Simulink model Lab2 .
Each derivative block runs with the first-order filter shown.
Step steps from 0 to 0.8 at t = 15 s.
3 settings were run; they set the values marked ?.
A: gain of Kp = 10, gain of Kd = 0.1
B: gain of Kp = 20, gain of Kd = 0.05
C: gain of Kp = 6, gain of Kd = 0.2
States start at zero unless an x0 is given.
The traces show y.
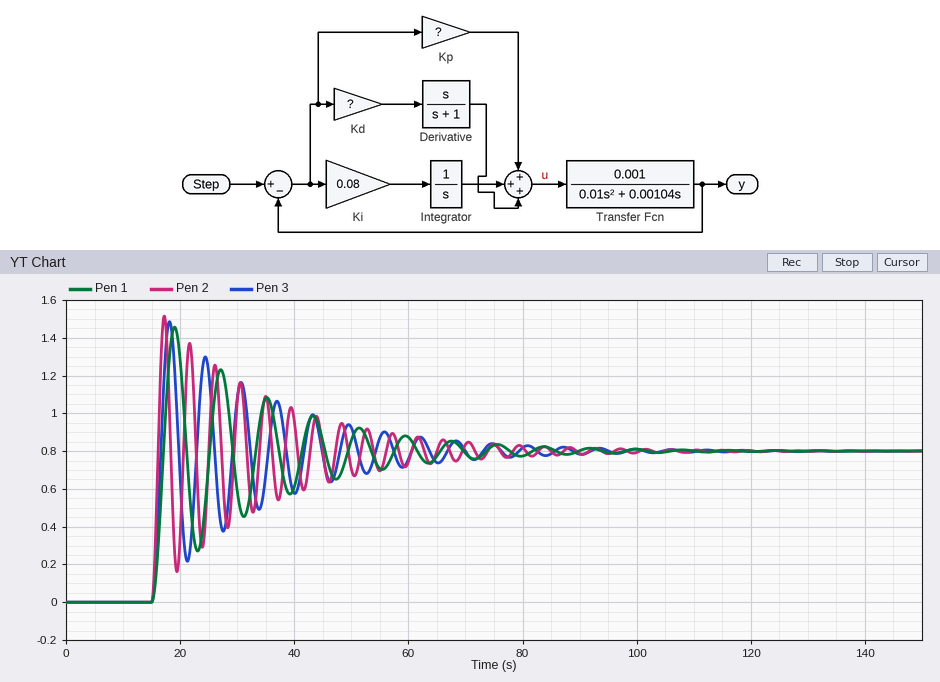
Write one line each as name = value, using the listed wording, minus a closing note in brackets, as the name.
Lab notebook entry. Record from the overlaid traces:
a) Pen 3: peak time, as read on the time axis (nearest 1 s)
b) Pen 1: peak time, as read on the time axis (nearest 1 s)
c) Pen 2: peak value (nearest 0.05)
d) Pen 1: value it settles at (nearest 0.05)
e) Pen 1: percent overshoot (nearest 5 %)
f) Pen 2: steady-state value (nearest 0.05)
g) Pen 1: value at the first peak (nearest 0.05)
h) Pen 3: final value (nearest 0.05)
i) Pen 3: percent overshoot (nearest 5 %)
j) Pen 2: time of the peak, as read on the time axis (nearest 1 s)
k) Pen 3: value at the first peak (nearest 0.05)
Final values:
Pen 3: peak time, as read on the time axis = 18 s
Pen 1: peak time, as read on the time axis = 19 s
Pen 2: peak value = 1.50
Pen 1: value it settles at = 0.80
Pen 1: percent overshoot = 80 %
Pen 2: steady-state value = 0.80
Pen 1: value at the first peak = 1.45
Pen 3: final value = 0.80
Pen 3: percent overshoot = 85 %
Pen 2: time of the peak, as read on the time axis = 17 s
Pen 3: value at the first peak = 1.50
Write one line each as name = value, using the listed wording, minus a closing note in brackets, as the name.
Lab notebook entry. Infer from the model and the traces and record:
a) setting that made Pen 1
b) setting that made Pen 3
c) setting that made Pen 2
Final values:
setting that made Pen 1 = C
setting that made Pen 3 = A
setting that made Pen 2 = B
